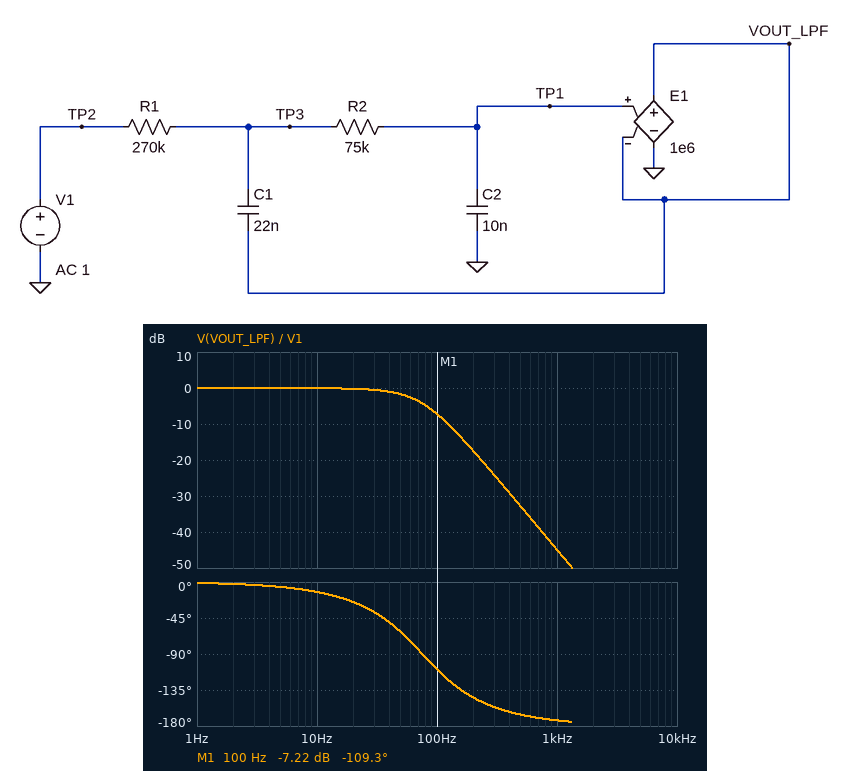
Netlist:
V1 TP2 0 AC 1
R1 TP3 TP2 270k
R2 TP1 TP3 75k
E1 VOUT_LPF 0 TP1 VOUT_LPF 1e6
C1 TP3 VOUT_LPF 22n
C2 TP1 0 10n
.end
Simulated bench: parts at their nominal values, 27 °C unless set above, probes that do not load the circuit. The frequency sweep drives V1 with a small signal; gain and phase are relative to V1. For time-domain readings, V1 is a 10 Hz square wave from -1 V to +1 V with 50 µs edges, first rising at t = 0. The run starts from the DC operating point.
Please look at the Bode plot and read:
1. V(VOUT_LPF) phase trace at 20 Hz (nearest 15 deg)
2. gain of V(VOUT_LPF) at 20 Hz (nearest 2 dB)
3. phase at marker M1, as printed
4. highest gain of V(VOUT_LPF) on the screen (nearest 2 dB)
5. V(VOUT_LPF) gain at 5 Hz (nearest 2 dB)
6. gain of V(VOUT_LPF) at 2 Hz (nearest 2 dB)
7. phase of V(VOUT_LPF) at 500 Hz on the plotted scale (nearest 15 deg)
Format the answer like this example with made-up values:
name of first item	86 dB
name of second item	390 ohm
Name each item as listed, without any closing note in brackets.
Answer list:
V(VOUT_LPF) phase trace at 20 Hz	-30 deg
gain of V(VOUT_LPF) at 20 Hz	0 dB
phase at marker M1, as printed	-109.3 deg
highest gain of V(VOUT_LPF) on the screen	0 dB
V(VOUT_LPF) gain at 5 Hz	0 dB
gain of V(VOUT_LPF) at 2 Hz	0 dB
phase of V(VOUT_LPF) at 500 Hz on the plotted scale	-165 deg
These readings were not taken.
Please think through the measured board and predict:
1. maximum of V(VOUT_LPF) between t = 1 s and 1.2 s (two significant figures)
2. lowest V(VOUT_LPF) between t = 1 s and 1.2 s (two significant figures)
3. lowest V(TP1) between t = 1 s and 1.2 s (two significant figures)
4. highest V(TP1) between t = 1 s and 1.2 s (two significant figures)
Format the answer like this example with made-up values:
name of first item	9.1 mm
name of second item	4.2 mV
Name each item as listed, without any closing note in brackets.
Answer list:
maximum of V(VOUT_LPF) between t = 1 s and 1.2 s	1.0 V
lowest V(VOUT_LPF) between t = 1 s and 1.2 s	-1.0 V
lowest V(TP1) between t = 1 s and 1.2 s	-1.0 V
highest V(TP1) between t = 1 s and 1.2 s	1.0 V
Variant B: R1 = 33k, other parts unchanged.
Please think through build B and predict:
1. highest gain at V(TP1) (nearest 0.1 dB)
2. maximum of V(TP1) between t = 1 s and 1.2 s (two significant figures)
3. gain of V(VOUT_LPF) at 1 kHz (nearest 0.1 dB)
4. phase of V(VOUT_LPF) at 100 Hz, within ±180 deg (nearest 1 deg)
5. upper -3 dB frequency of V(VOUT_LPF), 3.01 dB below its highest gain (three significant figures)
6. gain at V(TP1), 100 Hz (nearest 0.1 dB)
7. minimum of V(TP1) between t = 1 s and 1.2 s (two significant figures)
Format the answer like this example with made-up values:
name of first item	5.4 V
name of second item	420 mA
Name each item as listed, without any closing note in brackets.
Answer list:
highest gain at V(TP1)	0 dB
maximum of V(TP1) between t = 1 s and 1.2 s	1.1 V
gain of V(VOUT_LPF) at 1 kHz	-26.7 dB
phase of V(VOUT_LPF) at 100 Hz, within ±180 deg	-41 deg
upper -3 dB frequency of V(VOUT_LPF), 3.01 dB below its highest gain	208 Hz
gain at V(TP1), 100 Hz	-0.3 dB
minimum of V(TP1) between t = 1 s and 1.2 s	-1.1 V
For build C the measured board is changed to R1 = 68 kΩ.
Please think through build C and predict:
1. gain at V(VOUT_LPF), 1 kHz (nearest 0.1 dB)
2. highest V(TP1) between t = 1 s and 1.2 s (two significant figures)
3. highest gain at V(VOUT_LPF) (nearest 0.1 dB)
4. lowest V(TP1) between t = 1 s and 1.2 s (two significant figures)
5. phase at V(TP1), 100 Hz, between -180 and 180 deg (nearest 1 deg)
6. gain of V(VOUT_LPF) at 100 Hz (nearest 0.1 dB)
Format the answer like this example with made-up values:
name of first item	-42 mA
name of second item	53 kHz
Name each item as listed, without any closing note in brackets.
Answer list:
gain at V(VOUT_LPF), 1 kHz	-32.9 dB
highest V(TP1) between t = 1 s and 1.2 s	1.1 V
highest gain at V(VOUT_LPF)	0 dB
lowest V(TP1) between t = 1 s and 1.2 s	-1.1 V
phase at V(TP1), 100 Hz, between -180 and 180 deg	-58 deg
gain of V(VOUT_LPF) at 100 Hz	-0.5 dB
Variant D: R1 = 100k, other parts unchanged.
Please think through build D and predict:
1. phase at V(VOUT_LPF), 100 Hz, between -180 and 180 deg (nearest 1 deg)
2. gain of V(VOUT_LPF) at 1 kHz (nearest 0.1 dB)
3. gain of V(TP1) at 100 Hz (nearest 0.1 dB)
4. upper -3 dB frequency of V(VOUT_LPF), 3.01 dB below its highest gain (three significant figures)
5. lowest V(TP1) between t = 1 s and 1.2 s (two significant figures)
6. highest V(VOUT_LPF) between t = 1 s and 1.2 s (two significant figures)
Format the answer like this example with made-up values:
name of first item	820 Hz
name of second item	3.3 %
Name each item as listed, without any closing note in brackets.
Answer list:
phase at V(VOUT_LPF), 100 Hz, between -180 and 180 deg	-72 deg
gain of V(VOUT_LPF) at 1 kHz	-36.3 dB
gain of V(TP1) at 100 Hz	-1.2 dB
upper -3 dB frequency of V(VOUT_LPF), 3.01 dB below its highest gain	128 Hz
lowest V(TP1) between t = 1 s and 1.2 s	-1.1 V
highest V(VOUT_LPF) between t = 1 s and 1.2 s	1.1 V
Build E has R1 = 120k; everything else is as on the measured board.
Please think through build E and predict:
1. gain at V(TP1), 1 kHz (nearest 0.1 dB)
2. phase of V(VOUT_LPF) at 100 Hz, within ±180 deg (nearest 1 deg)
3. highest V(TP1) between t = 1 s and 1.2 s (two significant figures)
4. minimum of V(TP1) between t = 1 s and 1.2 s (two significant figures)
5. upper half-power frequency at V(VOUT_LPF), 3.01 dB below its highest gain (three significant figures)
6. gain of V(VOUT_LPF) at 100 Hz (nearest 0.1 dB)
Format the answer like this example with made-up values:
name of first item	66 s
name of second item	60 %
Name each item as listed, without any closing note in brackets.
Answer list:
gain at V(TP1), 1 kHz	-37.9 dB
phase of V(VOUT_LPF) at 100 Hz, within ±180 deg	-80 deg
highest V(TP1) between t = 1 s and 1.2 s	1.1 V
minimum of V(TP1) between t = 1 s and 1.2 s	-1.1 V
upper half-power frequency at V(VOUT_LPF), 3.01 dB below its highest gain	115 Hz
gain of V(VOUT_LPF) at 100 Hz	-1.9 dB
